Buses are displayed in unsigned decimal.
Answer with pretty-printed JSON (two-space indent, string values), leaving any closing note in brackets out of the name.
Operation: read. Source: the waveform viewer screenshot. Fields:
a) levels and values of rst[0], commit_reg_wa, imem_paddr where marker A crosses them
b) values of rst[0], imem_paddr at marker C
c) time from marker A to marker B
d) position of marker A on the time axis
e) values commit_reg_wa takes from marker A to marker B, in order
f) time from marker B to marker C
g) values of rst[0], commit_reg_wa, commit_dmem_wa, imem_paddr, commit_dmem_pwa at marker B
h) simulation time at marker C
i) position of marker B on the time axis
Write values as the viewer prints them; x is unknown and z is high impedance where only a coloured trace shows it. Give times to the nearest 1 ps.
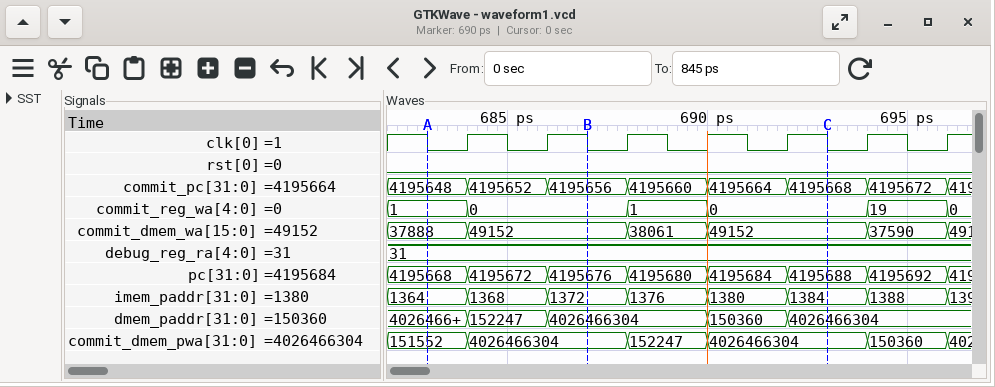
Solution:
{
  "levels and values of rst[0], commit_reg_wa, imem_paddr where marker A crosses them": "rst[0]=0, commit_reg_wa=1, imem_paddr=1364",
  "values of rst[0], imem_paddr at marker C": "rst[0]=0, imem_paddr=1384",
  "time from marker A to marker B": "4 ps",
  "position of marker A on the time axis": "683 ps",
  "values commit_reg_wa takes from marker A to marker B, in order": "1, 0",
  "time from marker B to marker C": "6 ps",
  "values of rst[0], commit_reg_wa, commit_dmem_wa, imem_paddr, commit_dmem_pwa at marker B": "rst[0]=0, commit_reg_wa=0, commit_dmem_wa=49152, imem_paddr=1372, commit_dmem_pwa=4026466304",
  "simulation time at marker C": "693 ps",
  "position of marker B on the time axis": "687 ps"
}
